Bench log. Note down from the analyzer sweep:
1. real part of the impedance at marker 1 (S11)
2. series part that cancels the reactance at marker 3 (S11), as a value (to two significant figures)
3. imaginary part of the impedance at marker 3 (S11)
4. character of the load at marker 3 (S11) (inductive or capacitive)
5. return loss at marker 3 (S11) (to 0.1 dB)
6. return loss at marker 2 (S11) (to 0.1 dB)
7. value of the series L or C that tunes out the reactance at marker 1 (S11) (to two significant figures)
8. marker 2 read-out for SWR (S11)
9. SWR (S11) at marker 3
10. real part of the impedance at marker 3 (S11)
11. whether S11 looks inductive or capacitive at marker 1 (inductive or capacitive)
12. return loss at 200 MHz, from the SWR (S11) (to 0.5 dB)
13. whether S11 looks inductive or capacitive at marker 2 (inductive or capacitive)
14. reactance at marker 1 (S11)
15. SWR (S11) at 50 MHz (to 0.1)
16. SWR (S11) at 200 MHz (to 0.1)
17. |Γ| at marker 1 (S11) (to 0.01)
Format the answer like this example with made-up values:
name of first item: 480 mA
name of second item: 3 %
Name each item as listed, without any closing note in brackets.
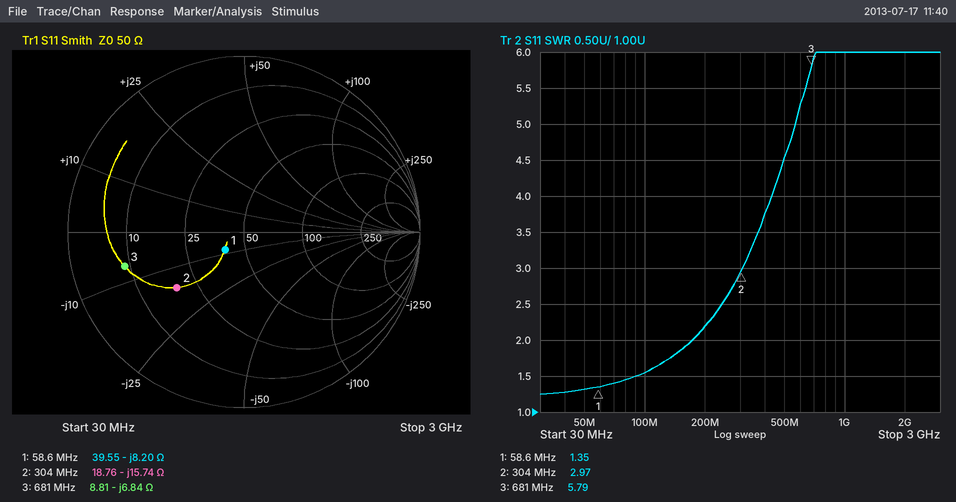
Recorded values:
real part of the impedance at marker 1: 39.55 Ω
series part that cancels the reactance at marker 3 (S11), as a value: 1.6 nH
imaginary part of the impedance at marker 3: -6.84 Ω
character of the load at marker 3 (S11): capacitive
return loss at marker 3 (S11): 3.0 dB
return loss at marker 2 (S11): 6.1 dB
value of the series L or C that tunes out the reactance at marker 1 (S11): 22 nH
marker 2 read-out for SWR: 2.97
SWR (S11) at marker 3: 5.79
real part of the impedance at marker 3: 8.81 Ω
whether S11 looks inductive or capacitive at marker 1: capacitive
return loss at 200 MHz, from the SWR (S11): 8.5 dB
whether S11 looks inductive or capacitive at marker 2: capacitive
reactance at marker 1: -8.20 Ω
SWR (S11) at 50 MHz: 1.3
SWR (S11) at 200 MHz: 2.2
|Γ| at marker 1 (S11): 0.15
